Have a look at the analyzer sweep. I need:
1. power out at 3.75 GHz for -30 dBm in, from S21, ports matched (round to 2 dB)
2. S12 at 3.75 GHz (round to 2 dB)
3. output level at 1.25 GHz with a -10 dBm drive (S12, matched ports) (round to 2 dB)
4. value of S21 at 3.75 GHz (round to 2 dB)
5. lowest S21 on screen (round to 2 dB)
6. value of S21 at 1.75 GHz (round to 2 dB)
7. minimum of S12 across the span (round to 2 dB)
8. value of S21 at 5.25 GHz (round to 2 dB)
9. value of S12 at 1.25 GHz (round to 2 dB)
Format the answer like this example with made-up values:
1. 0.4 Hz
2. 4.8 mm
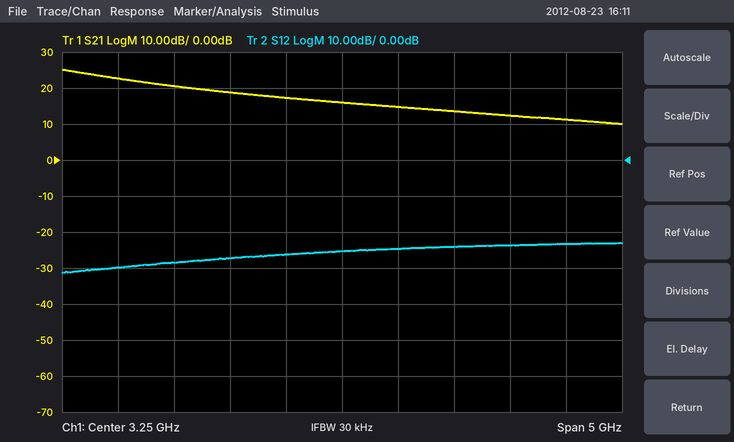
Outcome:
1. -16 dBm
2. -24 dB
3. -40 dBm
4. 14 dB
5. 10 dB
6. 20 dB
7. -32 dB
8. 12 dB
9. -30 dB
